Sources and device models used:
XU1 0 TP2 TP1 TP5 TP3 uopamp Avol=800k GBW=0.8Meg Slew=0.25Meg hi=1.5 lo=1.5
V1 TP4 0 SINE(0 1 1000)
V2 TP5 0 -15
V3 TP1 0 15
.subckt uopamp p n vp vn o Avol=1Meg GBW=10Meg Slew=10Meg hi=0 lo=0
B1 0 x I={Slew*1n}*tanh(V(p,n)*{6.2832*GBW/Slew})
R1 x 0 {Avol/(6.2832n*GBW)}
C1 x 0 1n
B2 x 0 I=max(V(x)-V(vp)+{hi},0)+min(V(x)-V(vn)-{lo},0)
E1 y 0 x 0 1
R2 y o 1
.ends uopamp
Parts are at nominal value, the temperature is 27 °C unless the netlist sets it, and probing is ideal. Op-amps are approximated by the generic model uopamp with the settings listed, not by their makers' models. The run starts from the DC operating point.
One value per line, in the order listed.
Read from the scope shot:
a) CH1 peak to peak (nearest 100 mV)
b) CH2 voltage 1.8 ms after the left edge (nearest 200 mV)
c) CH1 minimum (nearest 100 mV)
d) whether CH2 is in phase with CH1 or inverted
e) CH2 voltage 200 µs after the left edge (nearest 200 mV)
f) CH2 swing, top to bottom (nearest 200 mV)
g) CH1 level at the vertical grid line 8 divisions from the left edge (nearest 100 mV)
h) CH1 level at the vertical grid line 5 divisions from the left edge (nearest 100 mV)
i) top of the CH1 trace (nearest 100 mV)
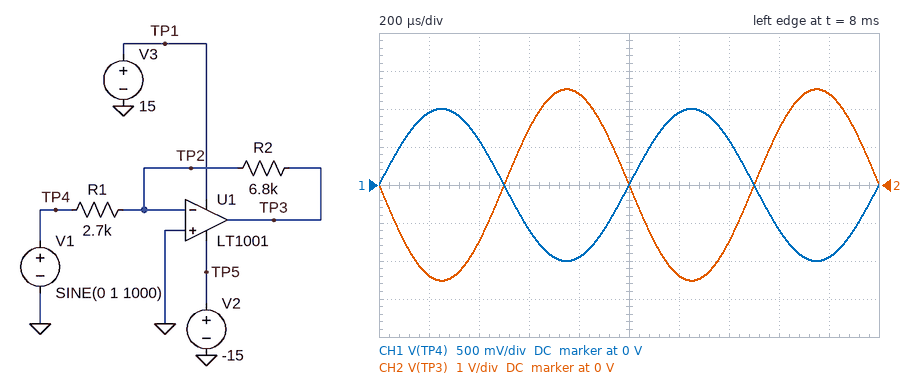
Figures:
2.0 V
2.4 V
-1.0 V
inverted
-2.4 V
5.0 V
-600 mV
0 V
1.0 V
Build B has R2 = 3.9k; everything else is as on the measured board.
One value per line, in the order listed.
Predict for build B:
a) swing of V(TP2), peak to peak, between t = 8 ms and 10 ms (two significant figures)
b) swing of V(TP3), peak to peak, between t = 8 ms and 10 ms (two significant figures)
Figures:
3.6 mV
2.9 V
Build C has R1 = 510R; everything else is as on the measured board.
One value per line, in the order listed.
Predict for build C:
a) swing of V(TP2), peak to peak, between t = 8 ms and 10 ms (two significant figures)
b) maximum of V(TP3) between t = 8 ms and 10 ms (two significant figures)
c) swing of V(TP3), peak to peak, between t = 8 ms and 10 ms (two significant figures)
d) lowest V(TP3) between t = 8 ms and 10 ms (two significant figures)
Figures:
35 mV
13 V
27 V
-13 V
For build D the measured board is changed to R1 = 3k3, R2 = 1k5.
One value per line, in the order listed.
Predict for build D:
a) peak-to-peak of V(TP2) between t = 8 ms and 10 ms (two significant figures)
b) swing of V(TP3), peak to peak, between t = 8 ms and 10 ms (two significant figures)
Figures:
1.1 mV
910 mV
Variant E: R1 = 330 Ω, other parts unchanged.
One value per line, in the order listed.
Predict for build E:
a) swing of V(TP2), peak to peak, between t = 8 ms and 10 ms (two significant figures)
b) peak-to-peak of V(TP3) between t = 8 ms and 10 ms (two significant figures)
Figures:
660 mV
27 V
